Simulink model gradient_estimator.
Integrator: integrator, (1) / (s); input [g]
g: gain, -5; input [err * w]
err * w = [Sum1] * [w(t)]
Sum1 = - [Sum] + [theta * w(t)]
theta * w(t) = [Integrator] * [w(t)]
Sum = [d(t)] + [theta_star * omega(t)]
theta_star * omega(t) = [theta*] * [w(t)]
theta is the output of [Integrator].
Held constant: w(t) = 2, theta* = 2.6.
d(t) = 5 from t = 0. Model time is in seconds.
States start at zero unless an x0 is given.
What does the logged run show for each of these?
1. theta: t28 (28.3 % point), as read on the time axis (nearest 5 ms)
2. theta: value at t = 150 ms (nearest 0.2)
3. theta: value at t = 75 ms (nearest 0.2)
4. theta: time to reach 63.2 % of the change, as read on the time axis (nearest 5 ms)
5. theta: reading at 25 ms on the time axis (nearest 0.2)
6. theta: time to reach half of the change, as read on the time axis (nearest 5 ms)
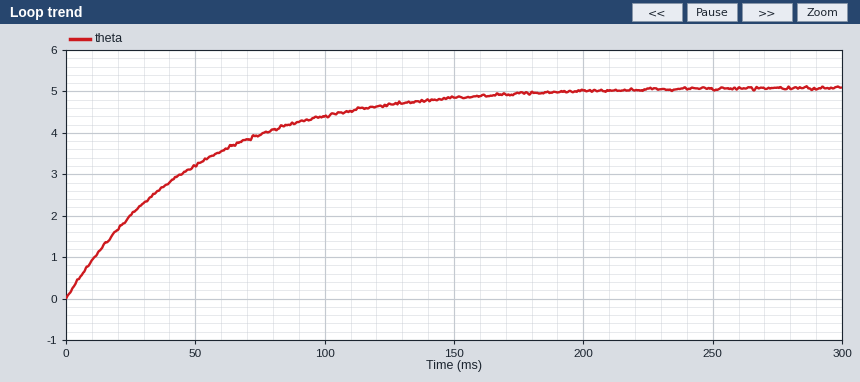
15 ms
4.8
4.0
50 ms
2.0
35 ms
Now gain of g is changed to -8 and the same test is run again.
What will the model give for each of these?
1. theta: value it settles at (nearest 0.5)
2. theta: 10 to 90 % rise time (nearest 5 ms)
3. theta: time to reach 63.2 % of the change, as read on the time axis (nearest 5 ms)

5.0
70 ms
30 ms
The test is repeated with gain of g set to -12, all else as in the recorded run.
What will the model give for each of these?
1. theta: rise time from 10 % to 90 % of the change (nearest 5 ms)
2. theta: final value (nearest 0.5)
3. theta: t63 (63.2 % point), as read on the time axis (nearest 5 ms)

45 ms
5.0
20 ms
